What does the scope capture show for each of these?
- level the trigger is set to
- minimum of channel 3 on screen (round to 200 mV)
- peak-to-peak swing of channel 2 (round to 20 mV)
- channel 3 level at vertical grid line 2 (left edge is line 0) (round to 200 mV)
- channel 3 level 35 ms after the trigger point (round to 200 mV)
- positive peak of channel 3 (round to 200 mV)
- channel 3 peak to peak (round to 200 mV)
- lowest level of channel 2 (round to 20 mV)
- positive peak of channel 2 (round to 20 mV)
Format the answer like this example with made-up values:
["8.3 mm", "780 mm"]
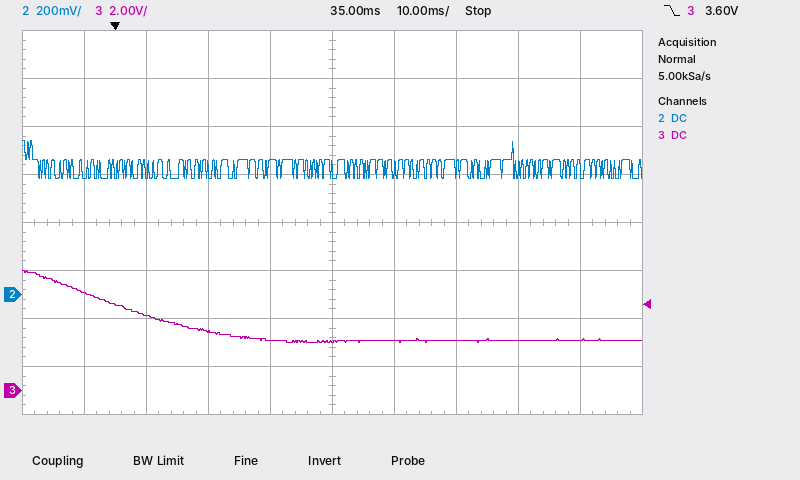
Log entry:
["3.60 V", "2.0 V", "160 mV", "3.2 V", "2.0 V", "5.0 V", "3.0 V", "480 mV", "640 mV"]
